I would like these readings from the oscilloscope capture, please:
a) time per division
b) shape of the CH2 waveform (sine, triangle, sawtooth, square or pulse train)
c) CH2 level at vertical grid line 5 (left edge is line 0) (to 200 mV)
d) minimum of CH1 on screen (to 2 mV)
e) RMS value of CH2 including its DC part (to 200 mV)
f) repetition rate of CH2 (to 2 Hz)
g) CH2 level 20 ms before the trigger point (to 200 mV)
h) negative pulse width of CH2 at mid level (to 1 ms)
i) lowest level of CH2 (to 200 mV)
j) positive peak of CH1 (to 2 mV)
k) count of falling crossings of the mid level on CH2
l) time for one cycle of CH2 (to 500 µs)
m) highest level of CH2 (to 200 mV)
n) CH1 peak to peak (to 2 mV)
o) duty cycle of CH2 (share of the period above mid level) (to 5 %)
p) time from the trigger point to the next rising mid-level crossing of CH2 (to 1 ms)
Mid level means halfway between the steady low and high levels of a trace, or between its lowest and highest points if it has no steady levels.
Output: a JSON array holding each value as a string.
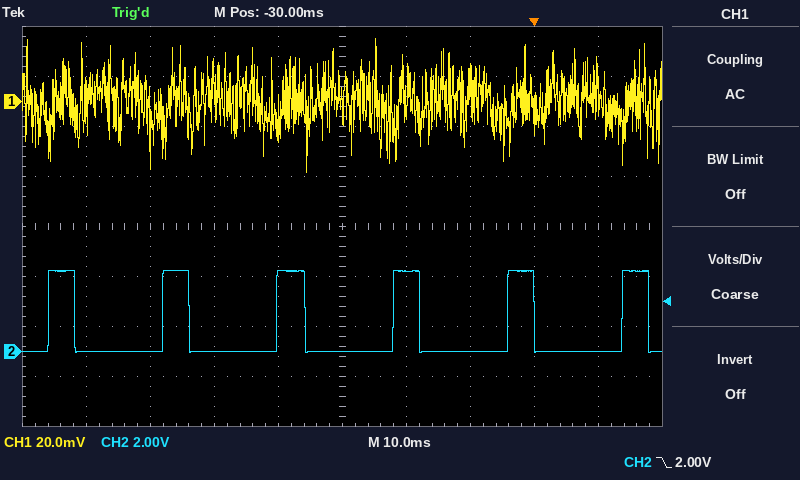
["10 ms", "pulse train", "0.0 V", "-28 mV", "1.6 V", "56 Hz", "3.2 V", "14 ms", "0.0 V", "26 mV", "6", "18.0 ms", "3.2 V", "54 mV", "25 %", "14 ms"]
